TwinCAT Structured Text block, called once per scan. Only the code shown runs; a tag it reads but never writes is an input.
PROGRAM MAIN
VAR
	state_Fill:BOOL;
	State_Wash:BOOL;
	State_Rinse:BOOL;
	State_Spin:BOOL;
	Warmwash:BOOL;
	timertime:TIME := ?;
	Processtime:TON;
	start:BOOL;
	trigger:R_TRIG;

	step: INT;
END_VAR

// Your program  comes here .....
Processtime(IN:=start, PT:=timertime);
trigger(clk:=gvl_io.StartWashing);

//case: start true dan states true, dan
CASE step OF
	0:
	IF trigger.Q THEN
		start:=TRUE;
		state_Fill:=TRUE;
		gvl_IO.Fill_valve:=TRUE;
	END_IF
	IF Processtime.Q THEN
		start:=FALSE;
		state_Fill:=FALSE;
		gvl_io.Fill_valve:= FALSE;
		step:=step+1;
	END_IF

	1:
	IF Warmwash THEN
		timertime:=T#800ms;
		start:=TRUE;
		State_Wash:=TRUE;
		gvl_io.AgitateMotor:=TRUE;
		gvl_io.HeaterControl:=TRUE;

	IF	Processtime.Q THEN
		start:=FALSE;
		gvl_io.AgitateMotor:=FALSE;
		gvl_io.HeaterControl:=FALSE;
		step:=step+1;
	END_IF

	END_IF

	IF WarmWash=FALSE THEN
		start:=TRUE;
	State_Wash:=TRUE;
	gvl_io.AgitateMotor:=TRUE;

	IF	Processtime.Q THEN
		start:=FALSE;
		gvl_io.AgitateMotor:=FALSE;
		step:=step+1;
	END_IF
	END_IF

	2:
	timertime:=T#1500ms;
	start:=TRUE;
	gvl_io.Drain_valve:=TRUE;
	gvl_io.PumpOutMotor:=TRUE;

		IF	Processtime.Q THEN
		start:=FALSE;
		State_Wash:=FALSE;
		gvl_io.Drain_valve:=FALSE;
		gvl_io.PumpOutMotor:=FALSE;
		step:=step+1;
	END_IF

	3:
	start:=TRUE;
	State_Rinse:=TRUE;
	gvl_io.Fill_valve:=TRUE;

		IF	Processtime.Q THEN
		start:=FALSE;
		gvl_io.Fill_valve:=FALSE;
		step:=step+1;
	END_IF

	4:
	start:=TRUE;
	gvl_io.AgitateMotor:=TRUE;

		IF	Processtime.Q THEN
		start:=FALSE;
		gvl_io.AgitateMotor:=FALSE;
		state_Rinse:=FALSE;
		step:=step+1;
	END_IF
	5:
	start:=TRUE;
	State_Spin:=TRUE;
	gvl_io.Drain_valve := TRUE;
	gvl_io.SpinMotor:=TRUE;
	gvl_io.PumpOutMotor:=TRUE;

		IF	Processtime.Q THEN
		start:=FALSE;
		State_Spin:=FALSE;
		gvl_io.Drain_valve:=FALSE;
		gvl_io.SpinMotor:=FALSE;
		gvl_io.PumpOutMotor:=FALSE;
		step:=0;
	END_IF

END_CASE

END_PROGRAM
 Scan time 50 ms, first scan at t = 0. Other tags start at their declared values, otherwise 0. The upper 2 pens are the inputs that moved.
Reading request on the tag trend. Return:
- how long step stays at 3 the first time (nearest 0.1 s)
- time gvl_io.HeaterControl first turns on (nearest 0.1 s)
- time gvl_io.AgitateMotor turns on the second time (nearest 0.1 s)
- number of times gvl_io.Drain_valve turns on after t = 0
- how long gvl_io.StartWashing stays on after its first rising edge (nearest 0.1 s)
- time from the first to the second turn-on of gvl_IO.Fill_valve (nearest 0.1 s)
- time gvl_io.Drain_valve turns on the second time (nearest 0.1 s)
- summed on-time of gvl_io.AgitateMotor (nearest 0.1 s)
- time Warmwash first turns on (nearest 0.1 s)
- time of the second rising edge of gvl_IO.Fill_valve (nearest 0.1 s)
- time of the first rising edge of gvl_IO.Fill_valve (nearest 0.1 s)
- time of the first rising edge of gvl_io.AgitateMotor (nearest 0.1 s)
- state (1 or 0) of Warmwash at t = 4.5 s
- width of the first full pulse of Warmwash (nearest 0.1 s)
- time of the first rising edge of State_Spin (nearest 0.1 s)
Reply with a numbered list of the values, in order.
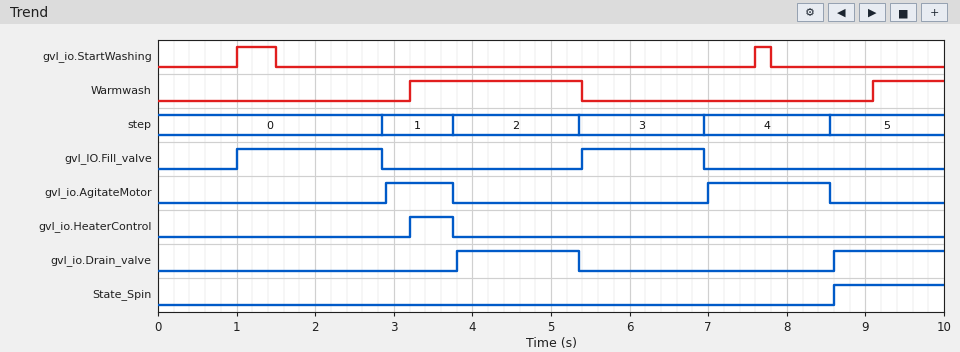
1. 1.6 s
2. 3.2 s
3. 7.0 s
4. 2
5. 0.5 s
6. 4.4 s
7. 8.6 s
8. 2.4 s
9. 3.2 s
10. 5.4 s
11. 1.0 s
12. 2.9 s
13. 1
14. 2.2 s
15. 8.6 s
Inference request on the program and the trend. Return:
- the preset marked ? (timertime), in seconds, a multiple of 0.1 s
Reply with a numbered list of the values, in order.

1. 1.8 s
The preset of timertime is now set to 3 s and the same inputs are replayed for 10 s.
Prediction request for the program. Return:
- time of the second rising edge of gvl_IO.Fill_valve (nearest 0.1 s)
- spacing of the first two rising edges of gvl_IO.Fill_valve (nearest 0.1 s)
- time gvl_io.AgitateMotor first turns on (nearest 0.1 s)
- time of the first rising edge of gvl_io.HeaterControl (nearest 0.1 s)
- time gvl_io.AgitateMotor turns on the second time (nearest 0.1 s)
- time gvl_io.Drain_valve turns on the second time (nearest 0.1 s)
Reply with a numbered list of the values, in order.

1. 6.6 s
2. 5.6 s
3. 4.1 s
4. 4.1 s
5. 8.2 s
6. 9.8 s
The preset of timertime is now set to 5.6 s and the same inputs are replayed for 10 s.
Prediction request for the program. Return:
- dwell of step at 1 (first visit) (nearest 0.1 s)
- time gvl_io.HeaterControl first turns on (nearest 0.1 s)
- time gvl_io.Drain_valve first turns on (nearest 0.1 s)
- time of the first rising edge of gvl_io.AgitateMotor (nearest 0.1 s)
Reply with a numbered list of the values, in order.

1. 2.5 s
2. 9.1 s
3. 9.2 s
4. 6.7 s
